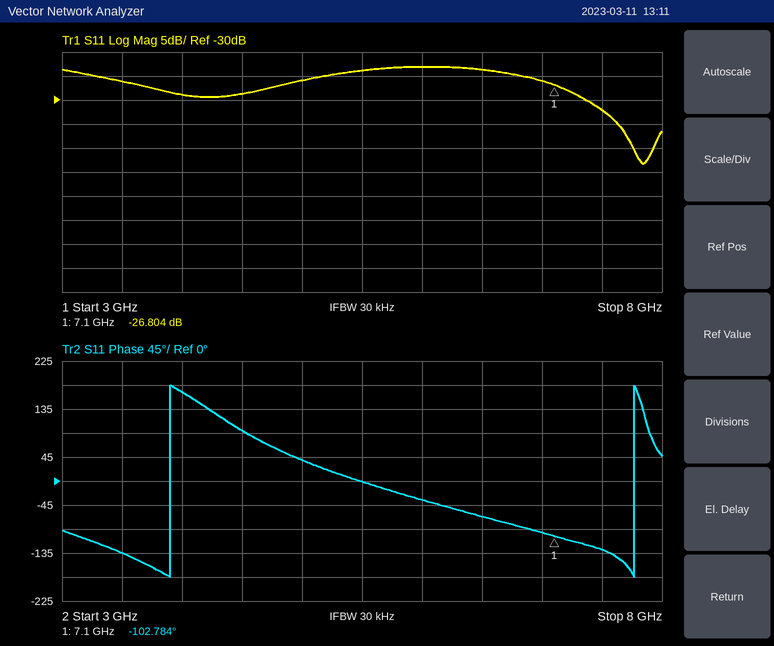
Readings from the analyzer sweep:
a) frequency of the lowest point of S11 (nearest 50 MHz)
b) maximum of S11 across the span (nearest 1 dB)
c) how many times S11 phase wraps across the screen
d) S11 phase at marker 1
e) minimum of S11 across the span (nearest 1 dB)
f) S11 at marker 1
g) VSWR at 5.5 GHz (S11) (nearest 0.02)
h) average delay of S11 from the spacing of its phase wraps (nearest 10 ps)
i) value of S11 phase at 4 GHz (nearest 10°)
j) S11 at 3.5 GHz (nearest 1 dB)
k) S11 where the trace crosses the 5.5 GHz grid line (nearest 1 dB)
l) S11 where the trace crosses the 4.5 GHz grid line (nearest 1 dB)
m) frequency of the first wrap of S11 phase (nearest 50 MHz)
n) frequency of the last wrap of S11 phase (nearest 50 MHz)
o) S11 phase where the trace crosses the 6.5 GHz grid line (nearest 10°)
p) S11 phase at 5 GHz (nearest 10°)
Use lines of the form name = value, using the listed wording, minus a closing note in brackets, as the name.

frequency of the lowest point of S11 = 7.85 GHz
maximum of S11 across the span = -23 dB
how many times S11 phase wraps across the screen = 2
S11 phase at marker 1 = -102.784°
minimum of S11 across the span = -43 dB
S11 at marker 1 = -26.804 dB
VSWR at 5.5 GHz (S11) = 1.14
average delay of S11 from the spacing of its phase wraps = 260 ps
value of S11 phase at 4 GHz = 170°
S11 at 3.5 GHz = -26 dB
S11 where the trace crosses the 5.5 GHz grid line = -24 dB
S11 where the trace crosses the 4.5 GHz grid line = -29 dB
frequency of the first wrap of S11 phase = 3.90 GHz
frequency of the last wrap of S11 phase = 7.75 GHz
S11 phase where the trace crosses the 6.5 GHz grid line = -70°
S11 phase at 5 GHz = 40°
